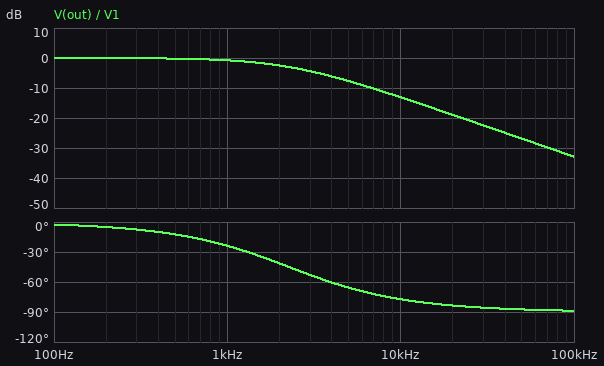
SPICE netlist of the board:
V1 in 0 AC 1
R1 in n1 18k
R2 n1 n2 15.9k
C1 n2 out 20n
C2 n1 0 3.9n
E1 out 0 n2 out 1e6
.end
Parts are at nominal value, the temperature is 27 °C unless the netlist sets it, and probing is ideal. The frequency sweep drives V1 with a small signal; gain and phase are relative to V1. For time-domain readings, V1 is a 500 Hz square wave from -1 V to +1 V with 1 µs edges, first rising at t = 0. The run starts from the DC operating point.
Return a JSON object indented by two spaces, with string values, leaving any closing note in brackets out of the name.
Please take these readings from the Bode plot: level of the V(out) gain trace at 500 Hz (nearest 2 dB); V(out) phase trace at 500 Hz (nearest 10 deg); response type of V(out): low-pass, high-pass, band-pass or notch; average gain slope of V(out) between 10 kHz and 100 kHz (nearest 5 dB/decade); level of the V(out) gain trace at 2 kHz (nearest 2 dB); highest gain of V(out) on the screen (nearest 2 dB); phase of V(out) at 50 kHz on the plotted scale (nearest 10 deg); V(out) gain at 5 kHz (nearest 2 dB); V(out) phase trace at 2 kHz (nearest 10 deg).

{
  "level of the V(out) gain trace at 500 Hz": "0 dB",
  "V(out) phase trace at 500 Hz": "-10 deg",
  "response type of V(out): low-pass, high-pass, band-pass or notch": "low-pass",
  "average gain slope of V(out) between 10 kHz and 100 kHz": "-20 dB/decade",
  "level of the V(out) gain trace at 2 kHz": "-2 dB",
  "highest gain of V(out) on the screen": "0 dB",
  "phase of V(out) at 50 kHz on the plotted scale": "-90 deg",
  "V(out) gain at 5 kHz": "-8 dB",
  "V(out) phase trace at 2 kHz": "-40 deg"
}
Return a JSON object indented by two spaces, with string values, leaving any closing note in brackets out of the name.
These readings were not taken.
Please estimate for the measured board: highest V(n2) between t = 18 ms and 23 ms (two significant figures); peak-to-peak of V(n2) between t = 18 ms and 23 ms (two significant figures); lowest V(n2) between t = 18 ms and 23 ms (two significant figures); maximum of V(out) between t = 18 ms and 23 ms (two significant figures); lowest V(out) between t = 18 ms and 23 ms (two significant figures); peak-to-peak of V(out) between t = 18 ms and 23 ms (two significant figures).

{
  "highest V(n2) between t = 18 ms and 23 ms": "1.0 V",
  "peak-to-peak of V(n2) between t = 18 ms and 23 ms": "2.0 V",
  "lowest V(n2) between t = 18 ms and 23 ms": "-1.0 V",
  "maximum of V(out) between t = 18 ms and 23 ms": "1.0 V",
  "lowest V(out) between t = 18 ms and 23 ms": "-1.0 V",
  "peak-to-peak of V(out) between t = 18 ms and 23 ms": "2.0 V"
}
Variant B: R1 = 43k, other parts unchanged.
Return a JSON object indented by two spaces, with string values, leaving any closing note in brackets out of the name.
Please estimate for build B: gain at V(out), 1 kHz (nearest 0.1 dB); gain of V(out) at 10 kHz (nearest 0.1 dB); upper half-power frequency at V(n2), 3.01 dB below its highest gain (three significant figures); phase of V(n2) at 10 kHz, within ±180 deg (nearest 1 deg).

{
  "gain at V(out), 1 kHz": "-3.2 dB",
  "gain of V(out) at 10 kHz": "-20.5 dB",
  "upper half-power frequency at V(n2), 3.01 dB below its highest gain": "949 Hz",
  "phase of V(n2) at 10 kHz, within ±180 deg": "-85 deg"
}
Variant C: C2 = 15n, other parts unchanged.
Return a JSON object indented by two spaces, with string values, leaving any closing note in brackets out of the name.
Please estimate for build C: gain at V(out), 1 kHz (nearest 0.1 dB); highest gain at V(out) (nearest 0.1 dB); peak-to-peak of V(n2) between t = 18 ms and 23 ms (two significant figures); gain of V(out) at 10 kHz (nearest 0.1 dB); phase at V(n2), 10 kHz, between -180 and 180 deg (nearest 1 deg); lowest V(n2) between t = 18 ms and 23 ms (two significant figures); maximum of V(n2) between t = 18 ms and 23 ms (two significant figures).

{
  "gain at V(out), 1 kHz": "-5.9 dB",
  "highest gain at V(out)": "0 dB",
  "peak-to-peak of V(n2) between t = 18 ms and 23 ms": "1.9 V",
  "gain of V(out) at 10 kHz": "-24.6 dB",
  "phase at V(n2), 10 kHz, between -180 and 180 deg": "-87 deg",
  "lowest V(n2) between t = 18 ms and 23 ms": "-950 mV",
  "maximum of V(n2) between t = 18 ms and 23 ms": "950 mV"
}
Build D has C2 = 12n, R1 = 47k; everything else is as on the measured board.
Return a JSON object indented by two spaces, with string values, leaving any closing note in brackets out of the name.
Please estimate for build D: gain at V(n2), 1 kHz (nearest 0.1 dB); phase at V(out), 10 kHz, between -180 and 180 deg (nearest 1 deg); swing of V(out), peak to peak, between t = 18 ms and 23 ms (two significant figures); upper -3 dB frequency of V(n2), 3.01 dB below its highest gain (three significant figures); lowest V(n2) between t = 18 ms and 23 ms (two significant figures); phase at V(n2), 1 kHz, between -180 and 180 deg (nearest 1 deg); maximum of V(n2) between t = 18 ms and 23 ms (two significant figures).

{
  "gain at V(n2), 1 kHz": "-11.3 dB",
  "phase at V(out), 10 kHz, between -180 and 180 deg": "-88 deg",
  "swing of V(out), peak to peak, between t = 18 ms and 23 ms": "1.4 V",
  "upper -3 dB frequency of V(n2), 3.01 dB below its highest gain": "282 Hz",
  "lowest V(n2) between t = 18 ms and 23 ms": "-710 mV",
  "phase at V(n2), 1 kHz, between -180 and 180 deg": "-74 deg",
  "maximum of V(n2) between t = 18 ms and 23 ms": "710 mV"
}
